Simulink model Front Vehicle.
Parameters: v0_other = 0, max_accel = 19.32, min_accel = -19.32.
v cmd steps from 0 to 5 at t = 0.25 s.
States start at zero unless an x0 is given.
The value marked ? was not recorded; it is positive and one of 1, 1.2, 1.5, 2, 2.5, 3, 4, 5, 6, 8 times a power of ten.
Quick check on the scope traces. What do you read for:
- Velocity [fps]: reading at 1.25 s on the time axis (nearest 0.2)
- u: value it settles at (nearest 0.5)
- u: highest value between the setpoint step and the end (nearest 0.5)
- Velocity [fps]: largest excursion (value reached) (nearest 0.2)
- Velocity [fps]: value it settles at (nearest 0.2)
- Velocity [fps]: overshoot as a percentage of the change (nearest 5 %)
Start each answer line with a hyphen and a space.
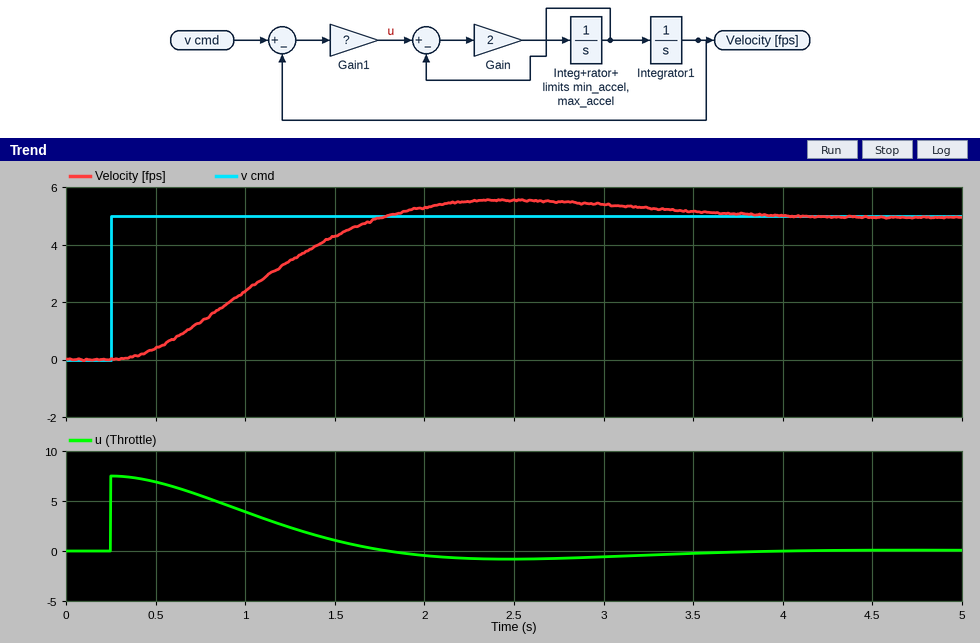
- 3.4
- 0.0
- 7.5
- 5.6
- 5.0
- 10 %
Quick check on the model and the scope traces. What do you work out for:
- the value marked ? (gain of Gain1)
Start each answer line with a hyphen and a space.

- 1.5
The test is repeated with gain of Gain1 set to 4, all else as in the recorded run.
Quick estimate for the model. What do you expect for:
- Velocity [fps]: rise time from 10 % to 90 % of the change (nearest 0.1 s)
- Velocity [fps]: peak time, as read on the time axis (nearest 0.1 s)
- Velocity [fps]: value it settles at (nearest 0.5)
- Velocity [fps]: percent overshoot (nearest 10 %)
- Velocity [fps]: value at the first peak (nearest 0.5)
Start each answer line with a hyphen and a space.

- 0.5 s
- 1.4 s
- 5.0
- 30 %
- 6.5
